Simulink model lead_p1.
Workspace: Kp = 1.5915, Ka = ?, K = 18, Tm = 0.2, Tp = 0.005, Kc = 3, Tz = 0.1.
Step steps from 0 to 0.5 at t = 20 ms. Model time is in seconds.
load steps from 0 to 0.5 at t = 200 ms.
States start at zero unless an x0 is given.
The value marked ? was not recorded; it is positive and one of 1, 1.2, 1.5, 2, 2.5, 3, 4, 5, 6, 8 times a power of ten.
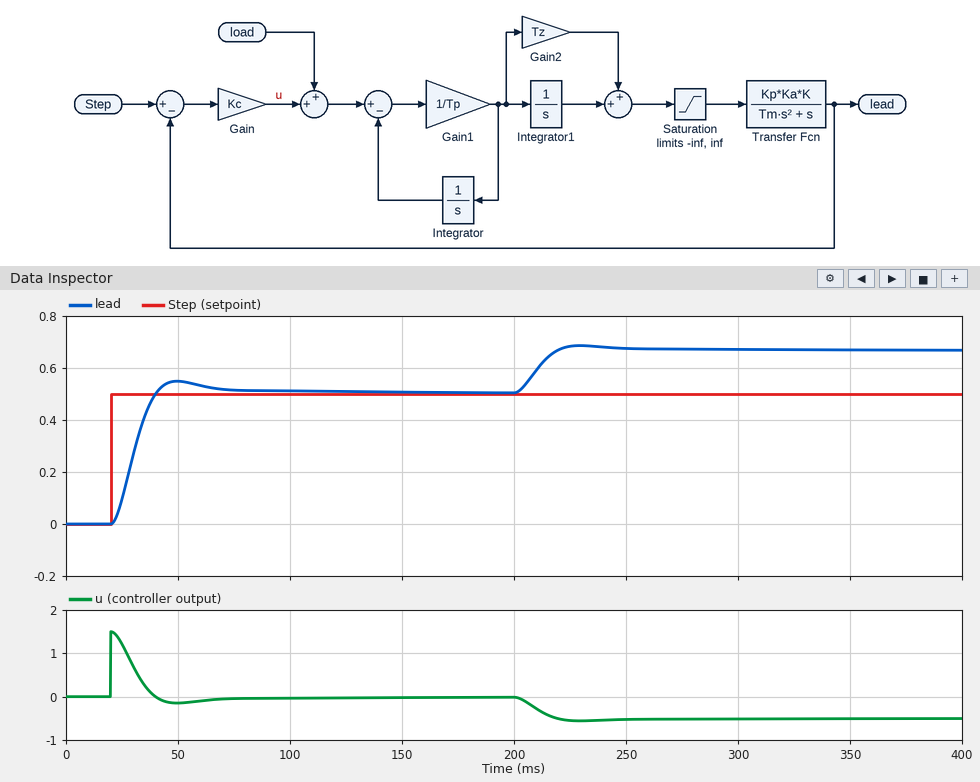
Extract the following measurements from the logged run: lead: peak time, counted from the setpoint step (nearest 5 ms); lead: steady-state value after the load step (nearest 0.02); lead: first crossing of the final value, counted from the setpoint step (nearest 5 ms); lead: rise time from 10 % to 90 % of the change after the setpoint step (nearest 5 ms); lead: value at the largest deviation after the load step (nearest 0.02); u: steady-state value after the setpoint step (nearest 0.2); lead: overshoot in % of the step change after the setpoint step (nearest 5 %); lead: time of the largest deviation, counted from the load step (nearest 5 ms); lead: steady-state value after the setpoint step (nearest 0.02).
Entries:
30 ms
0.66
20 ms
15 ms
0.68
0.0
10 %
30 ms
0.50
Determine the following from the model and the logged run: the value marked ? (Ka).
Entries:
2.5
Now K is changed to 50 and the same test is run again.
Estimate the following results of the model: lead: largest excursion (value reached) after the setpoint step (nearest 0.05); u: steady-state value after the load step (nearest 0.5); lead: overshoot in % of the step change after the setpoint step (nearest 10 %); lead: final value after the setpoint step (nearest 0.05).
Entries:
0.65
-0.5
30 %
0.50
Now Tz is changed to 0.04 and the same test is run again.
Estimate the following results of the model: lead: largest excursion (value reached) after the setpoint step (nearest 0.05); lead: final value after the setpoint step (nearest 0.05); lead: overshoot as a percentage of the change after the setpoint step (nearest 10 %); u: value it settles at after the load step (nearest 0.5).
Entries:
0.60
0.50
20 %
-0.5
